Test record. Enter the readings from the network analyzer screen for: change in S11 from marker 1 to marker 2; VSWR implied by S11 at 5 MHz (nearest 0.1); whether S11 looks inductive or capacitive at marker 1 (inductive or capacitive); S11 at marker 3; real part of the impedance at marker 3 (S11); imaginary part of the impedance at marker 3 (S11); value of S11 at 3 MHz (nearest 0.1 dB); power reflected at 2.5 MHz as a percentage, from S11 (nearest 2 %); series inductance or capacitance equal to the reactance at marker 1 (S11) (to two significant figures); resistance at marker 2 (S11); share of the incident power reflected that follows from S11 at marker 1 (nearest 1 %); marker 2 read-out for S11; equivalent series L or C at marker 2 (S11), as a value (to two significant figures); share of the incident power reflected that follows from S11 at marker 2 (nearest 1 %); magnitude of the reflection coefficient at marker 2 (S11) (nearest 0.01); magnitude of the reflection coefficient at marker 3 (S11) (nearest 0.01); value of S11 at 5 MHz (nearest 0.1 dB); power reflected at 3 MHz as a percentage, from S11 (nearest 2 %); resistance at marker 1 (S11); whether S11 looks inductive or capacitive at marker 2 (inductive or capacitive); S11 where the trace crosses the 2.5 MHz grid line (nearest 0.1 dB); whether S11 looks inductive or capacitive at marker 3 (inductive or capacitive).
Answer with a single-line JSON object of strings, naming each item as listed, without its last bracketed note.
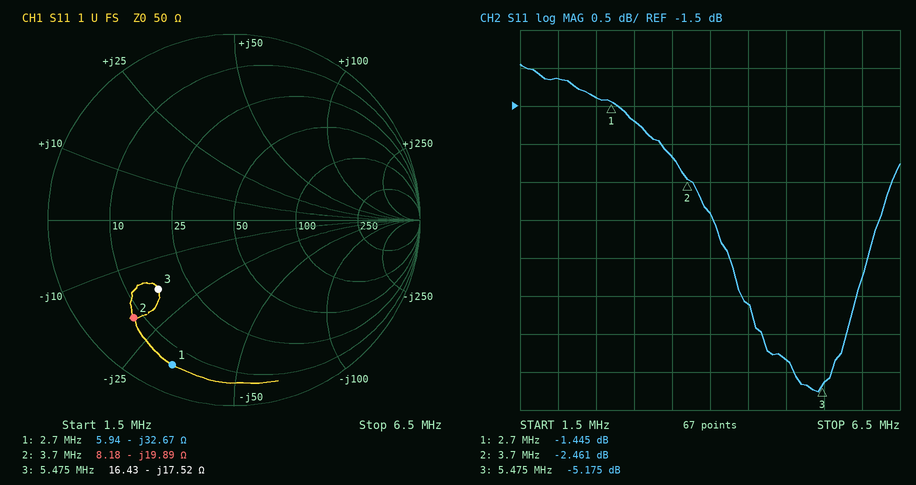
{"change in S11 from marker 1 to marker 2": "-1.016 dB", "VSWR implied by S11 at 5 MHz": "3.7", "whether S11 looks inductive or capacitive at marker 1": "capacitive", "S11 at marker 3": "-5.175 dB", "real part of the impedance at marker 3": "16.43 Ω", "imaginary part of the impedance at marker 3": "-17.52 Ω", "value of S11 at 3 MHz": "-1.7 dB", "power reflected at 2.5 MHz as a percentage, from S11": "72 %", "series inductance or capacitance equal to the reactance at marker 1 (S11)": "1.8 nF", "resistance at marker 2": "8.18 Ω", "share of the incident power reflected that follows from S11 at marker 1": "72 %", "marker 2 read-out for S11": "-2.461 dB", "equivalent series L or C at marker 2 (S11), as a value": "2.2 nF", "share of the incident power reflected that follows from S11 at marker 2": "57 %", "magnitude of the reflection coefficient at marker 2 (S11)": "0.75", "magnitude of the reflection coefficient at marker 3 (S11)": "0.55", "value of S11 at 5 MHz": "-4.8 dB", "power reflected at 3 MHz as a percentage, from S11": "68 %", "resistance at marker 1": "5.94 Ω", "whether S11 looks inductive or capacitive at marker 2": "capacitive", "S11 where the trace crosses the 2.5 MHz grid line": "-1.4 dB", "whether S11 looks inductive or capacitive at marker 3": "capacitive"}
